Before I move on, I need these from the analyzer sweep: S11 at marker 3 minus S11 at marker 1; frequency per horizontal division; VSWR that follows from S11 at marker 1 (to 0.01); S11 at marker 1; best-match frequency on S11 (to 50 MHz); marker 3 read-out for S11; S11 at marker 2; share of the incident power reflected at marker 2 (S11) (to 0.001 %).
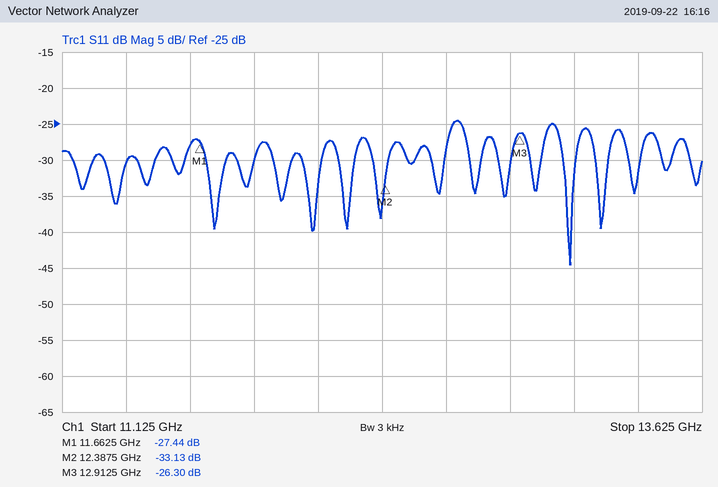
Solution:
1.14 dB
250 MHz
1.09
-27.44 dB
13.10 GHz
-26.30 dB
-33.13 dB
0.049 %
